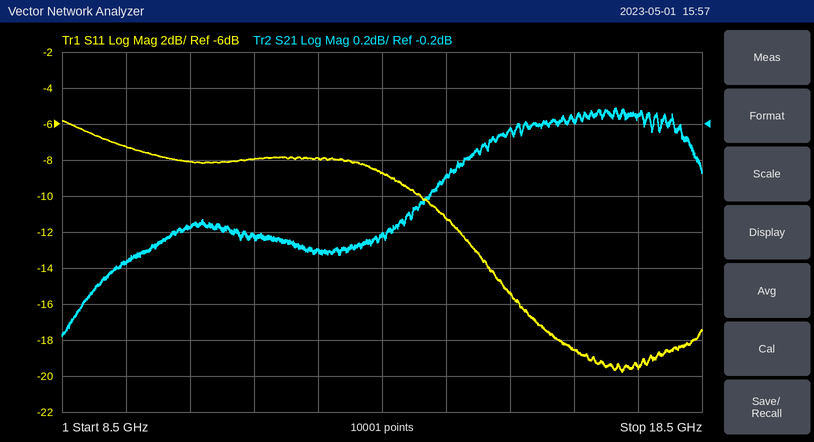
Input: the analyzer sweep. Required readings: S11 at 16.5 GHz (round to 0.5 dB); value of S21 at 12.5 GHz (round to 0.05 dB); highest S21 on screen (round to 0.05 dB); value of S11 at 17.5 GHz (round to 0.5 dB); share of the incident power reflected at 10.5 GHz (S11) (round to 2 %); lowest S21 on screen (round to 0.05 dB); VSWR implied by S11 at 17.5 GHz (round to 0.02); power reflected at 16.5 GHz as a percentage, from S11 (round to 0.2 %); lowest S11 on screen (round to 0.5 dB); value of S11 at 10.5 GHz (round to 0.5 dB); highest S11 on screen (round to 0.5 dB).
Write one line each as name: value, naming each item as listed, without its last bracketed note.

S11 at 16.5 GHz: -18.5 dB
value of S21 at 12.5 GHz: -0.90 dB
highest S21 on screen: -0.10 dB
value of S11 at 17.5 GHz: -19.5 dB
share of the incident power reflected at 10.5 GHz (S11): 16 %
lowest S21 on screen: -1.40 dB
VSWR implied by S11 at 17.5 GHz: 1.24
power reflected at 16.5 GHz as a percentage, from S11: 1.4 %
lowest S11 on screen: -20.0 dB
value of S11 at 10.5 GHz: -8.0 dB
highest S11 on screen: -6.0 dB
